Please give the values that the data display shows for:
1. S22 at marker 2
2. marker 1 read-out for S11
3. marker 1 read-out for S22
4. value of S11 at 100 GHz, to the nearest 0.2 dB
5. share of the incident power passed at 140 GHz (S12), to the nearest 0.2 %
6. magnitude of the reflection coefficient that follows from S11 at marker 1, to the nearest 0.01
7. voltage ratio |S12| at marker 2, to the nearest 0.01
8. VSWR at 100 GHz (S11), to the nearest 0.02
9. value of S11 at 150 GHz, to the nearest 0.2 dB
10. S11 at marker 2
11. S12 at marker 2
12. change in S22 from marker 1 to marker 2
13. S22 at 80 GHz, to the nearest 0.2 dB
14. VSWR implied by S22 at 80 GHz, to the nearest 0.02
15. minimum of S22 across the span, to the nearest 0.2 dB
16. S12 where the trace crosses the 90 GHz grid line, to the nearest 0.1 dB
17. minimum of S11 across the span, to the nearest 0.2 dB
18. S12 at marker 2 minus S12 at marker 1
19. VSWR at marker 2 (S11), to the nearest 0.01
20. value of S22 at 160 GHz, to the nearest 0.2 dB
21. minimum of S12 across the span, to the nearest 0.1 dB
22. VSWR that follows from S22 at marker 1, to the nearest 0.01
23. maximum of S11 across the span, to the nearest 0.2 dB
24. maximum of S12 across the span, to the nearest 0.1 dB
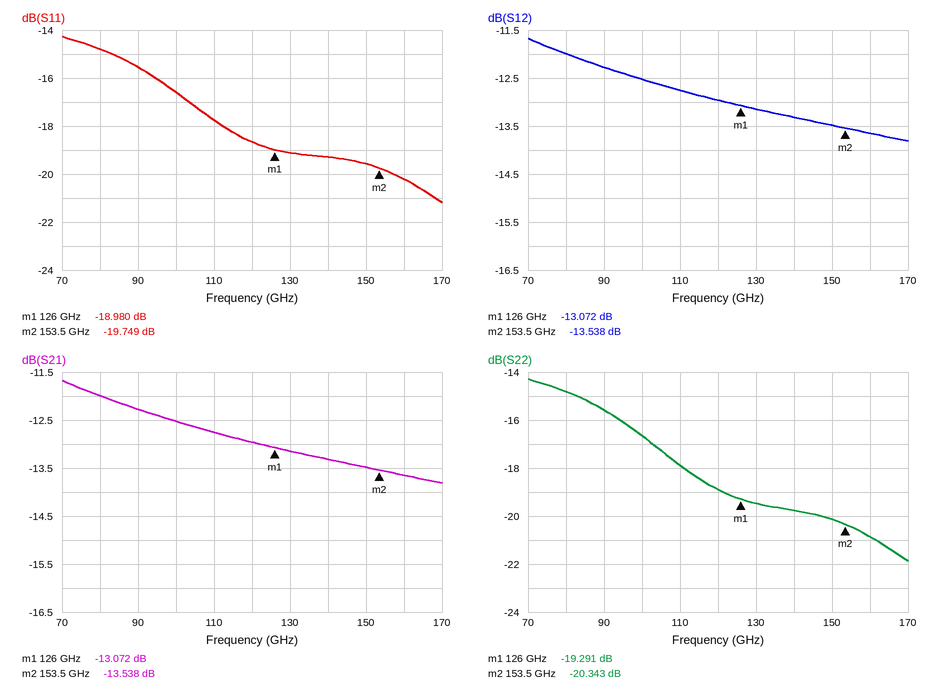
-20.343 dB
-18.980 dB
-19.291 dB
-16.6 dB
4.6 %
0.11
0.21
1.34
-19.6 dB
-19.749 dB
-13.538 dB
-1.052 dB
-14.8 dB
1.44
-21.8 dB
-12.3 dB
-21.2 dB
-0.466 dB
1.23
-20.8 dB
-13.8 dB
1.24
-14.2 dB
-11.7 dB
